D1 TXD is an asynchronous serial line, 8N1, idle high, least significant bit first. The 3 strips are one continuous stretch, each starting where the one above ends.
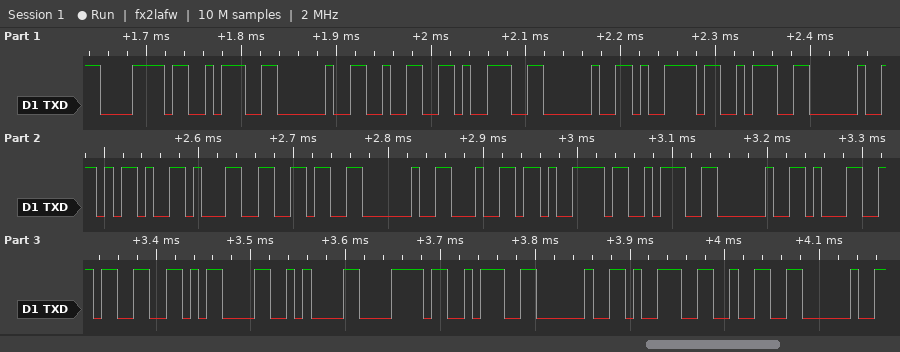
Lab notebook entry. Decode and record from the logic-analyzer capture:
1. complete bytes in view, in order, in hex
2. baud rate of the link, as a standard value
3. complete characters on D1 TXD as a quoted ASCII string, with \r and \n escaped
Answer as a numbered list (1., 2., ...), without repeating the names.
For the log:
1. 0x78 0x3A 0x20 0x32 0x39 0x20 0x79 0x3A 0x20 0x2D 0x31 0x36 0x20 0x64 0x79 0x3A 0x20 0x31 0x33 0x0D 0x0A 0x78 0x3A 0x20 0x39 0x32 0x20
2. 115200 baud
3. "x: 29 y: -16 dy: 13\r\nx: 92 "
